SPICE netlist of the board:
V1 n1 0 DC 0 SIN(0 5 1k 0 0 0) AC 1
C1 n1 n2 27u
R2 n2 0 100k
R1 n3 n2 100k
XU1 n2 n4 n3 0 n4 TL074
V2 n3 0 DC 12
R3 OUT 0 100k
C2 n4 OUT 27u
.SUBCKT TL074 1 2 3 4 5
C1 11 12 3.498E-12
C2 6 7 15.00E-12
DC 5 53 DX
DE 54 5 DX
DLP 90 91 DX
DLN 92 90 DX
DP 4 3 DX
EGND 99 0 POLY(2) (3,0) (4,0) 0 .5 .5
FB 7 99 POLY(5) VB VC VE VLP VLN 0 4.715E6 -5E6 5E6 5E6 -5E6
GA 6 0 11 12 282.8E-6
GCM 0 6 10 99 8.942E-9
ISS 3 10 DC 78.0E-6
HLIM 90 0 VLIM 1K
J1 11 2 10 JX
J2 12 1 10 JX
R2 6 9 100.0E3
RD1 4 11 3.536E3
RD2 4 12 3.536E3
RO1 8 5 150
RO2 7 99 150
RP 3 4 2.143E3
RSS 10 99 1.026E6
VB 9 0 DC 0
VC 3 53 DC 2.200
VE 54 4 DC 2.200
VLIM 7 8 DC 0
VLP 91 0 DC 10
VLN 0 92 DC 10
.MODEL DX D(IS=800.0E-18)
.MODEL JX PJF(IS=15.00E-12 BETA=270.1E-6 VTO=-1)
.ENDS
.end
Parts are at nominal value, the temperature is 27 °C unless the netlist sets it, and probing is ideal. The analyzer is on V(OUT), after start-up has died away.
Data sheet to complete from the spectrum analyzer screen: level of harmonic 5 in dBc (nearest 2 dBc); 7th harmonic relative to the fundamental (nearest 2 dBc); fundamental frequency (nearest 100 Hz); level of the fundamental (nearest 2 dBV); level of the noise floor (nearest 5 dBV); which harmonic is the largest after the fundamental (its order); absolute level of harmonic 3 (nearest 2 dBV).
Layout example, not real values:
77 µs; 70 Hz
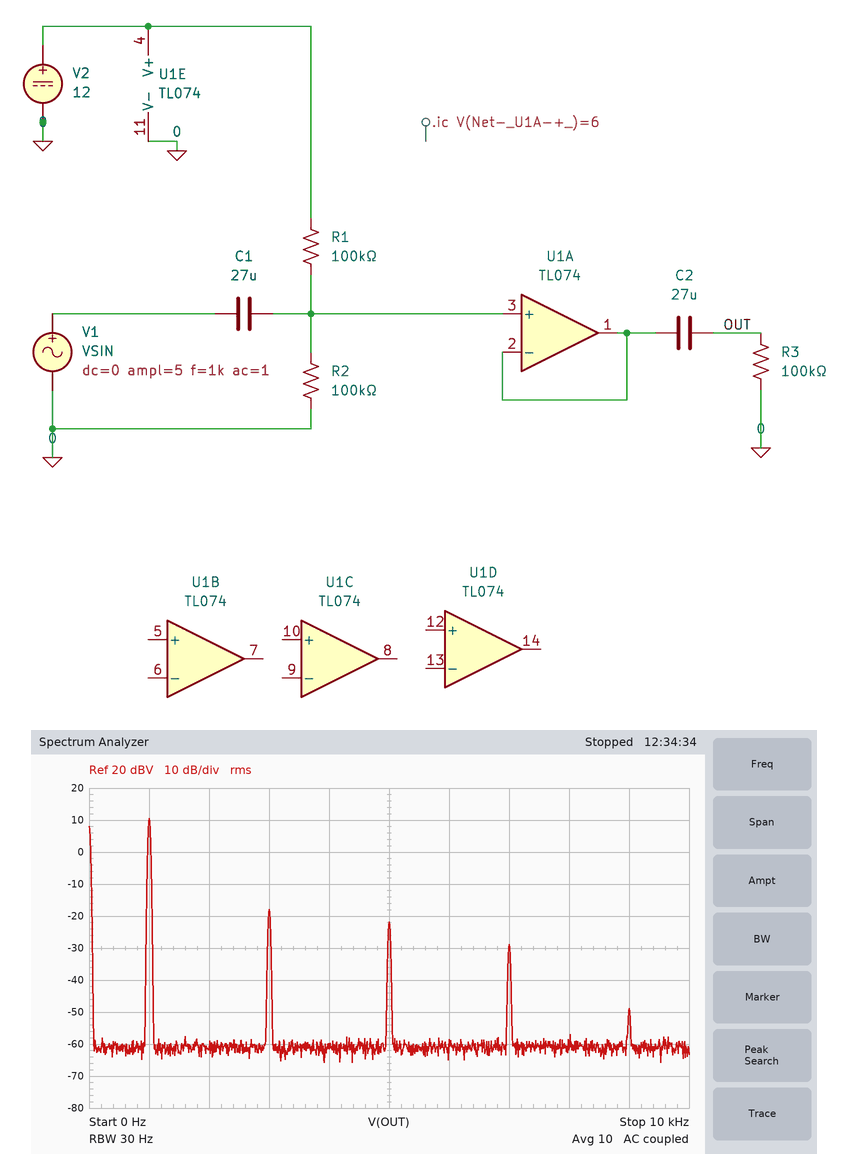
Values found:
-32 dBc; -40 dBc; 1.0 kHz; 10 dBV; -60 dBV; 3; -18 dBV
